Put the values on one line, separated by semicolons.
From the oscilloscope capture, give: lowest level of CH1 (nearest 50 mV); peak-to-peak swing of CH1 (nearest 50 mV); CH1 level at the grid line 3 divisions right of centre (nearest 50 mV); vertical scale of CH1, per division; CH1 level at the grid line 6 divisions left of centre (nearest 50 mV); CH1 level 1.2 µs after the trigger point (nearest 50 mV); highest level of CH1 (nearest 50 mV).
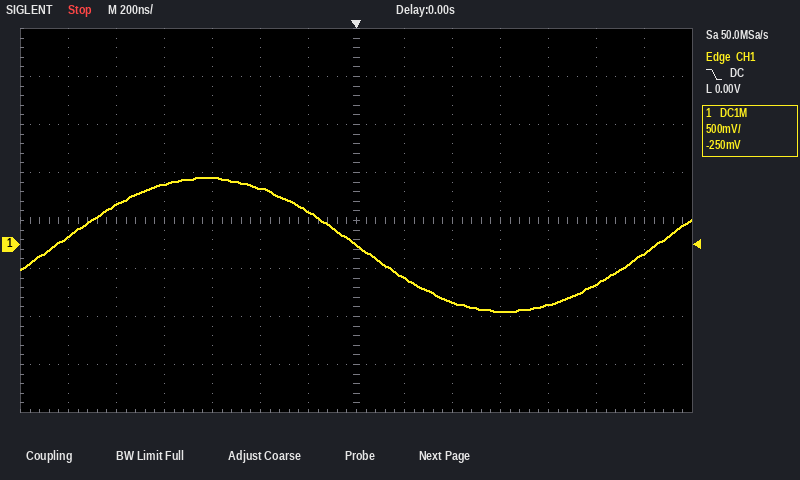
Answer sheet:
-700 mV; 1.40 V; -700 mV; 500 mV; 100 mV; -100 mV; 700 mV
